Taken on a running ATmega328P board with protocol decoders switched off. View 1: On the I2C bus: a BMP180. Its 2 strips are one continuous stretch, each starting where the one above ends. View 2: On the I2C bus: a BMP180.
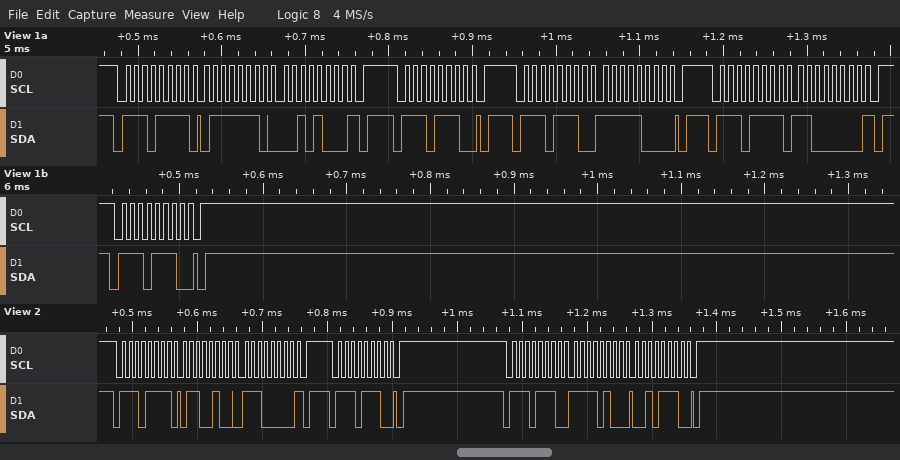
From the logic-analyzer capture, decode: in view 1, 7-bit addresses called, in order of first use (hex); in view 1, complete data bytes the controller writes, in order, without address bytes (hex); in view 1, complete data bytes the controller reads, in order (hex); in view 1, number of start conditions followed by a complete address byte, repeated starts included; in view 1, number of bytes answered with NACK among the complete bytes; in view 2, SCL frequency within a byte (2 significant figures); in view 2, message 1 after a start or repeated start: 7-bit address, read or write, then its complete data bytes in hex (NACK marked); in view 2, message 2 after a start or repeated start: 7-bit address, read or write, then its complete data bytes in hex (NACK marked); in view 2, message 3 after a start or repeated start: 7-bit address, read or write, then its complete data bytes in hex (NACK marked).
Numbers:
0x77
F8
7E 28 C0
5
2
100 kHz
0x77 read: 64 E0 NACK
0x77 write
0x77 write: F4 2E
